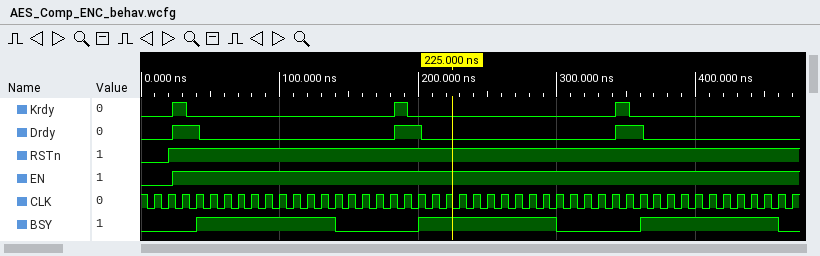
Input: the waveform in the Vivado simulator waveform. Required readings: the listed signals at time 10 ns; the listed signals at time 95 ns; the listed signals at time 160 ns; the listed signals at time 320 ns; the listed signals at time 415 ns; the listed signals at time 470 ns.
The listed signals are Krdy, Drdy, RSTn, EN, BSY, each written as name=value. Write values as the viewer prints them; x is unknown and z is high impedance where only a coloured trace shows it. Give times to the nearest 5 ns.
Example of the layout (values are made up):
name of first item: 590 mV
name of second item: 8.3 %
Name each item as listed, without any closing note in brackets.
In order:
the listed signals at time 10 ns: Krdy=0, Drdy=0, RSTn=0, EN=0, BSY=0
the listed signals at time 95 ns: Krdy=0, Drdy=0, RSTn=1, EN=1, BSY=1
the listed signals at time 160 ns: Krdy=0, Drdy=0, RSTn=1, EN=1, BSY=0
the listed signals at time 320 ns: Krdy=0, Drdy=0, RSTn=1, EN=1, BSY=0
the listed signals at time 415 ns: Krdy=0, Drdy=0, RSTn=1, EN=1, BSY=1
the listed signals at time 470 ns: Krdy=0, Drdy=0, RSTn=1, EN=1, BSY=0
